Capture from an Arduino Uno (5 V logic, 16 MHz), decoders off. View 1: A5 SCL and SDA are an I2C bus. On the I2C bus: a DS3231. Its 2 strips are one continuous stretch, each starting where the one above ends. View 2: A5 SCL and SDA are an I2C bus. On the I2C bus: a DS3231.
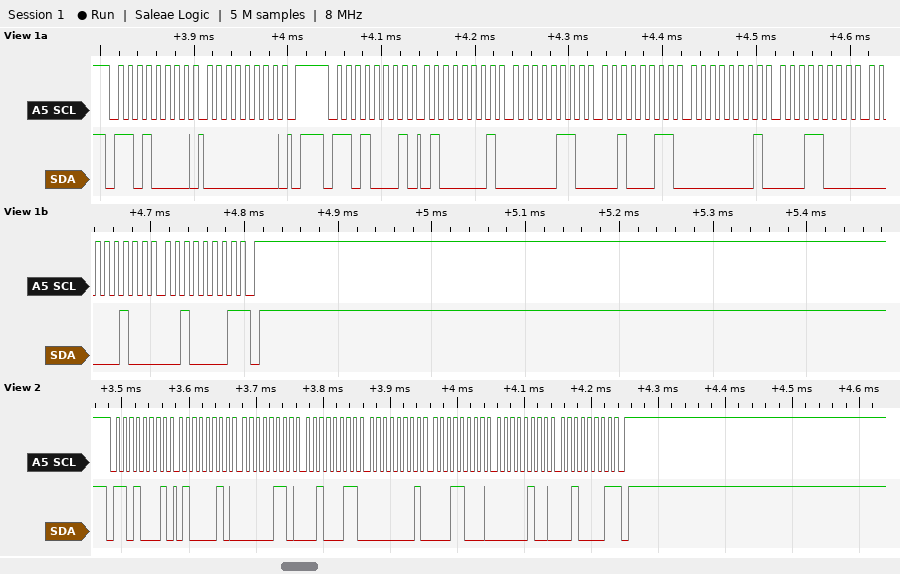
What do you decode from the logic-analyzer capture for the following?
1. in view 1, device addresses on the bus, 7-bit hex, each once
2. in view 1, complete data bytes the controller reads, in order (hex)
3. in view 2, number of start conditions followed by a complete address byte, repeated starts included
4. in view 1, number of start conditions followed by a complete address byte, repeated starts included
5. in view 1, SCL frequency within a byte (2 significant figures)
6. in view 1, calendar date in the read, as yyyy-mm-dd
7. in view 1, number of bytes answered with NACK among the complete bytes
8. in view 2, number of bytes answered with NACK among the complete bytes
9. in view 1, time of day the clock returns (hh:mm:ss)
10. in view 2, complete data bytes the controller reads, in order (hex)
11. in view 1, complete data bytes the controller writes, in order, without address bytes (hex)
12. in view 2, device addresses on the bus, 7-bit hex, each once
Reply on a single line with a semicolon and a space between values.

0x68; 41 06 23 01 18 04 21; 1; 2; 100 kHz; 2021-04-18; 1; 1; 23:06:41; 42 06 23 01 18 04 21; 00; 0x68
